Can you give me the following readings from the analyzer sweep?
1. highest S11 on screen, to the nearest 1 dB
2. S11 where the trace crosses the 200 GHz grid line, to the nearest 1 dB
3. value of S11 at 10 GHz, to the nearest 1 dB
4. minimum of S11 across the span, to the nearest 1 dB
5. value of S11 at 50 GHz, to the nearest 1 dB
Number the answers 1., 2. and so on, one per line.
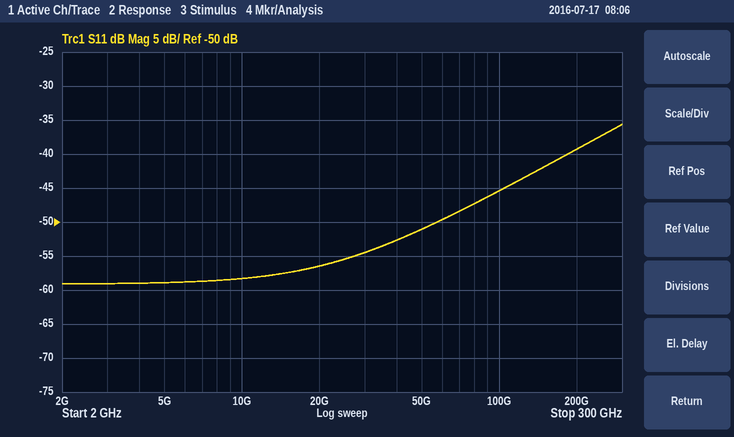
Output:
1. -36 dB
2. -39 dB
3. -58 dB
4. -59 dB
5. -51 dB
